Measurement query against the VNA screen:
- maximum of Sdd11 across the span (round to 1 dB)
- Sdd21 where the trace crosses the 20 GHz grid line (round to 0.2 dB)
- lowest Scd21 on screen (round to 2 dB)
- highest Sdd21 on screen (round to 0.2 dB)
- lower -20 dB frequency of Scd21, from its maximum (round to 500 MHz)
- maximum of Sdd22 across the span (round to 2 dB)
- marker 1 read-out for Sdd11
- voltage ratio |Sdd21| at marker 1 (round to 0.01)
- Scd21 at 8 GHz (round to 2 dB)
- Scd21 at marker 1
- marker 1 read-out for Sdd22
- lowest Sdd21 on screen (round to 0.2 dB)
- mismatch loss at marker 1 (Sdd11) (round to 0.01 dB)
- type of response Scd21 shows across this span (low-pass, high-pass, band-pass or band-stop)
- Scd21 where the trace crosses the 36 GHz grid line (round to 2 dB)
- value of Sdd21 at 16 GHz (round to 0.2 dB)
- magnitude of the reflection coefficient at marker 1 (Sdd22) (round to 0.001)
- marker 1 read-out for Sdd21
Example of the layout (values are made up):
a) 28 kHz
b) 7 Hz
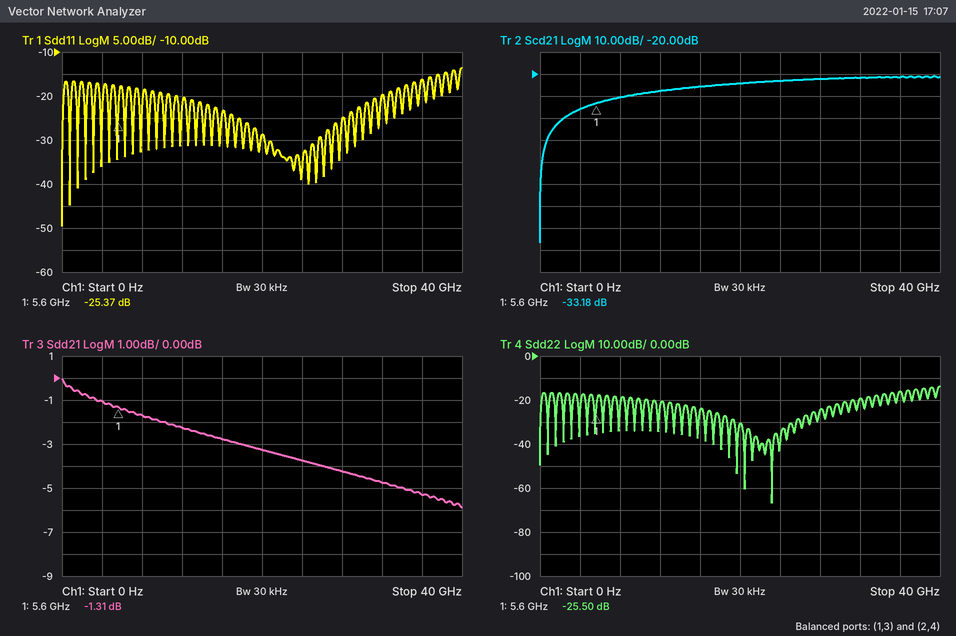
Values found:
a) -14 dB
b) -3.2 dB
c) -96 dB
d) 0.0 dB
e) 2.0 GHz
f) -14 dB
g) -25.37 dB
h) 0.86
i) -30 dB
j) -33.18 dB
k) -25.50 dB
l) -5.8 dB
m) 0.01 dB
n) high-pass
o) -22 dB
p) -2.8 dB
q) 0.053
r) -1.31 dB
